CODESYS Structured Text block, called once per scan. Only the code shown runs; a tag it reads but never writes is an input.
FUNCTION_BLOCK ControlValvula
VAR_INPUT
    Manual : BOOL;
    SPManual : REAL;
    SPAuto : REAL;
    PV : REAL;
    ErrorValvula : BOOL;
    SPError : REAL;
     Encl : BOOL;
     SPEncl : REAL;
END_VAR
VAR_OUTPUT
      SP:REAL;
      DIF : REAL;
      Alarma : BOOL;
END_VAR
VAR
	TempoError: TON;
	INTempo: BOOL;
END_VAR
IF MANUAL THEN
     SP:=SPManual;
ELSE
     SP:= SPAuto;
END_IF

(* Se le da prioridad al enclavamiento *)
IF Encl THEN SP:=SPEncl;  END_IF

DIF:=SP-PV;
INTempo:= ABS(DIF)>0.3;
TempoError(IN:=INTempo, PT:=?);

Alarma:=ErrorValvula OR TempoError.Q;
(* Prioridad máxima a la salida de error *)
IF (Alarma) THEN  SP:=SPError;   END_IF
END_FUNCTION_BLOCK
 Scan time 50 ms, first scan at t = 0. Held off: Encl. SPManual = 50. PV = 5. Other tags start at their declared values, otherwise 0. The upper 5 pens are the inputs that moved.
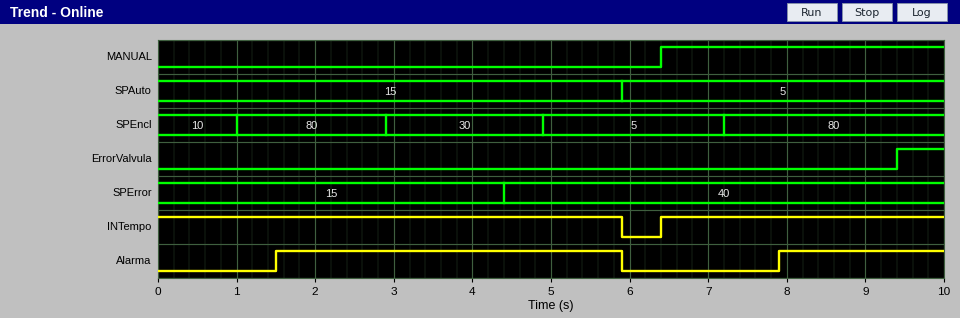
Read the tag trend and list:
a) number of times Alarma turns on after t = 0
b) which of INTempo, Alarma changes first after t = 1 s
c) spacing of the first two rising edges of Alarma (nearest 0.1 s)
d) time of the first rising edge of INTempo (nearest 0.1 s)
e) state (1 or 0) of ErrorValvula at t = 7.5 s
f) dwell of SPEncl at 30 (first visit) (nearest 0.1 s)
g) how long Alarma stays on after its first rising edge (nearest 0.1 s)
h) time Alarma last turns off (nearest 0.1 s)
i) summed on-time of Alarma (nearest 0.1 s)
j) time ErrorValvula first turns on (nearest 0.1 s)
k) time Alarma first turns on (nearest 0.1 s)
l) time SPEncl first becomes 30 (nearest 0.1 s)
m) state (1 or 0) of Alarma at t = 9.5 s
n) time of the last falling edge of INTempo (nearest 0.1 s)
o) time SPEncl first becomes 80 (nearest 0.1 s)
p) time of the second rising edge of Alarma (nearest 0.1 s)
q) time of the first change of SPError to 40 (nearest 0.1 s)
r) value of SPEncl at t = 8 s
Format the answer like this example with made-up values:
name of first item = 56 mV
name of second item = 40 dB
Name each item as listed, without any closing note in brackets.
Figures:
number of times Alarma turns on after t = 0 = 2
which of INTempo, Alarma changes first after t = 1 s = Alarma
spacing of the first two rising edges of Alarma = 6.4 s
time of the first rising edge of INTempo = 6.4 s
state (1 or 0) of ErrorValvula at t = 7.5 s = 0
dwell of SPEncl at 30 (first visit) = 2.0 s
how long Alarma stays on after its first rising edge = 4.4 s
time Alarma last turns off = 5.9 s
summed on-time of Alarma = 6.5 s
time ErrorValvula first turns on = 9.4 s
time Alarma first turns on = 1.5 s
time SPEncl first becomes 30 = 2.9 s
state (1 or 0) of Alarma at t = 9.5 s = 1
time of the last falling edge of INTempo = 5.9 s
time SPEncl first becomes 80 = 1.0 s
time of the second rising edge of Alarma = 7.9 s
time of the first change of SPError to 40 = 4.4 s
value of SPEncl at t = 8 s = 80
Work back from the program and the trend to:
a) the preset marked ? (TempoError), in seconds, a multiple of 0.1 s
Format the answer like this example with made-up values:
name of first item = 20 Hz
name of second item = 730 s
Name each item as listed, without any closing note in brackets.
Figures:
the preset marked ? (TempoError), in seconds, a multiple of 0.1 s = 1.5 s
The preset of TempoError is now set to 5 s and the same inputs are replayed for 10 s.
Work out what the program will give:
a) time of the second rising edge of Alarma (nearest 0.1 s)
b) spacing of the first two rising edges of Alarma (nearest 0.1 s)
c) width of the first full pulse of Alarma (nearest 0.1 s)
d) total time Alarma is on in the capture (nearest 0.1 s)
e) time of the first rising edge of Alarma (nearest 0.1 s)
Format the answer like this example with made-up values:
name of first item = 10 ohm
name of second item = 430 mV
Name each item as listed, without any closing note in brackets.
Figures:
time of the second rising edge of Alarma = 9.4 s
spacing of the first two rising edges of Alarma = 4.4 s
width of the first full pulse of Alarma = 0.9 s
total time Alarma is on in the capture = 1.5 s
time of the first rising edge of Alarma = 5.0 s
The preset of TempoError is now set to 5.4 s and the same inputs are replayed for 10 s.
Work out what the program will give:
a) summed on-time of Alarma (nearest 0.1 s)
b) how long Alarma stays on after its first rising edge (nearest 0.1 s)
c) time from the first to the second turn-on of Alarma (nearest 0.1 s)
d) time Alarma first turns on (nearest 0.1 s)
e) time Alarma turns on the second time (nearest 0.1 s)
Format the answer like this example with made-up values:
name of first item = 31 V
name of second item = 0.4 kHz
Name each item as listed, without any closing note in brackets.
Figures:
summed on-time of Alarma = 1.1 s
how long Alarma stays on after its first rising edge = 0.5 s
time from the first to the second turn-on of Alarma = 4.0 s
time Alarma first turns on = 5.4 s
time Alarma turns on the second time = 9.4 s
